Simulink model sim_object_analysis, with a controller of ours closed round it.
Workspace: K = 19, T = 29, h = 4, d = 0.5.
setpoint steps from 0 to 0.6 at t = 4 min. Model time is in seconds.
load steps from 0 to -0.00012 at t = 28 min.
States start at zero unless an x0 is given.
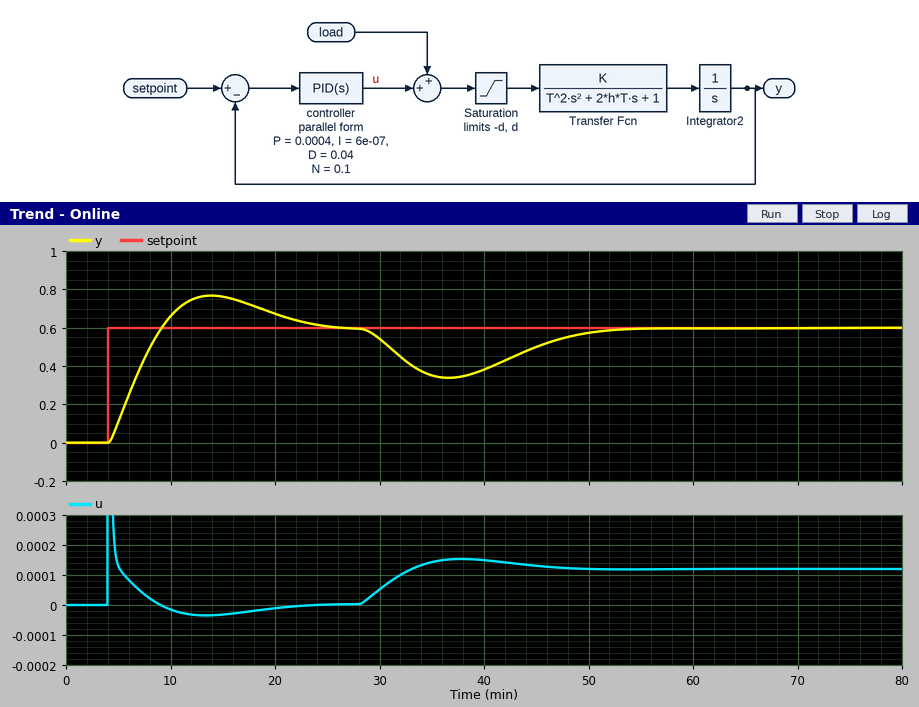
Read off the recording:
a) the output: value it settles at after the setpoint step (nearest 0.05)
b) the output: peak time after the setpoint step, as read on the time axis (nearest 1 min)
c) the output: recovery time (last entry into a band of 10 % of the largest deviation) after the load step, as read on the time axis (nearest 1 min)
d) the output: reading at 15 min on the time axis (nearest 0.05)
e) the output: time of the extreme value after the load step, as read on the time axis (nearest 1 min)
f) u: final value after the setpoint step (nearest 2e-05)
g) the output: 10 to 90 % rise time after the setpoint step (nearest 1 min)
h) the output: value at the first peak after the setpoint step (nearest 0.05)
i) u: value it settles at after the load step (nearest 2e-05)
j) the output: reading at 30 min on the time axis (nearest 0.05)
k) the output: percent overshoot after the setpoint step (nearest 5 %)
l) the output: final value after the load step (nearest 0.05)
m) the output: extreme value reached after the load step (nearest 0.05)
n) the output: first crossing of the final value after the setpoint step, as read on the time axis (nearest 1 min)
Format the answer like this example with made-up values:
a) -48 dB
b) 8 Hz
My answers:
a) 0.60
b) 14 min
c) 50 min
d) 0.75
e) 37 min
f) 0.00000
g) 4 min
h) 0.75
i) 0.00012
j) 0.55
k) 30 %
l) 0.60
m) 0.35
n) 9 min
